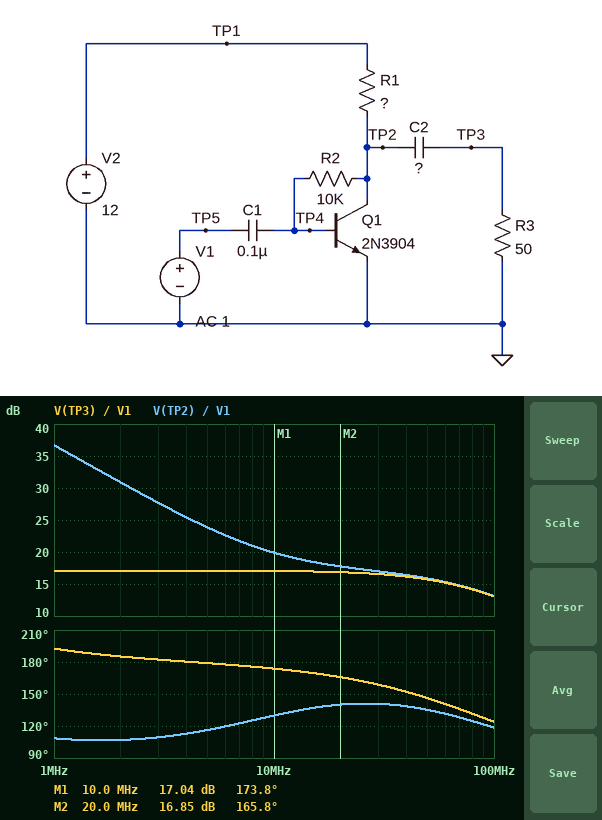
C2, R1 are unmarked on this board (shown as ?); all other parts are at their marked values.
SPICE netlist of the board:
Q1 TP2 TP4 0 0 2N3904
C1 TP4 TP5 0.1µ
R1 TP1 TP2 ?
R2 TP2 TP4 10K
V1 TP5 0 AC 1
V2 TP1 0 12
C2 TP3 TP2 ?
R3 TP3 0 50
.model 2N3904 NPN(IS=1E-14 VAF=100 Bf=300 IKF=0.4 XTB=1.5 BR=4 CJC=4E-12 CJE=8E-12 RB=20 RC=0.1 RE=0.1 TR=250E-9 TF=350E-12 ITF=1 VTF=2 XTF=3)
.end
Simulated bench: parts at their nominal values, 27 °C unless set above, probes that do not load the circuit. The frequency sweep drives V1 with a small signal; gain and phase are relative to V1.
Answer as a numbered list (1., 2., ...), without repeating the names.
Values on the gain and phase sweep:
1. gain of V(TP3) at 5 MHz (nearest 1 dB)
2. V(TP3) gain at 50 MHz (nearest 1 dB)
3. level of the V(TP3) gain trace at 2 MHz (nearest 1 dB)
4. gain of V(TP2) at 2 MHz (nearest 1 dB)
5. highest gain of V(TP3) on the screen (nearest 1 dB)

1. 17 dB
2. 16 dB
3. 17 dB
4. 31 dB
5. 17 dB
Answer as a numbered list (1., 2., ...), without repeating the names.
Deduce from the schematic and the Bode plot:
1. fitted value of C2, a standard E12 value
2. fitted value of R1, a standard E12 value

1. 330 pF
2. 2.7 kΩ
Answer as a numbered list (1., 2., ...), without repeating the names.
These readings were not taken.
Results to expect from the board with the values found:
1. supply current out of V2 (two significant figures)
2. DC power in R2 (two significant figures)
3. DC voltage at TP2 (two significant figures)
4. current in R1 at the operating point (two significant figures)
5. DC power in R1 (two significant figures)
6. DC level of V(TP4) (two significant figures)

1. 4.1 mA
2. 1.9 µW
3. 830 mV
4. 4.1 mA
5. 46 mW
6. 690 mV
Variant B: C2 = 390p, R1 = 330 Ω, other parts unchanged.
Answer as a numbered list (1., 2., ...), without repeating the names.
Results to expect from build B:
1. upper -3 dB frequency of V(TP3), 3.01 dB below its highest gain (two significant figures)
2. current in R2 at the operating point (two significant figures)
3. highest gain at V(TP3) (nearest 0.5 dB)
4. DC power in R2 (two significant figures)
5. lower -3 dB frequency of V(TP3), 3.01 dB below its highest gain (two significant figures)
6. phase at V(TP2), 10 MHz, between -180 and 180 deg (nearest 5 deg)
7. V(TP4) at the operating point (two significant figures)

1. 21 MHz
2. 110 µA
3. 30.5 dB
4. 120 µW
5. 940 kHz
6. 120 deg
7. 750 mV
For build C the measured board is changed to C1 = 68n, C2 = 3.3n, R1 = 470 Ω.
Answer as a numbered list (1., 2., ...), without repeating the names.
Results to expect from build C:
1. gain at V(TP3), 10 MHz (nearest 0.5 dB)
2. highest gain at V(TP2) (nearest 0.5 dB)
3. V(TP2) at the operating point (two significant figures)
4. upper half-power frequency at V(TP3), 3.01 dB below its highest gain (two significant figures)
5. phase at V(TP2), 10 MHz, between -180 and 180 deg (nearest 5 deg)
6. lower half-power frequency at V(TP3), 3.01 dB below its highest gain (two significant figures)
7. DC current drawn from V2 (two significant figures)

1. 29.0 dB
2. 48.0 dB
3. 1.5 V
4. 22 MHz
5. 150 deg
6. 84 kHz
7. 22 mA
